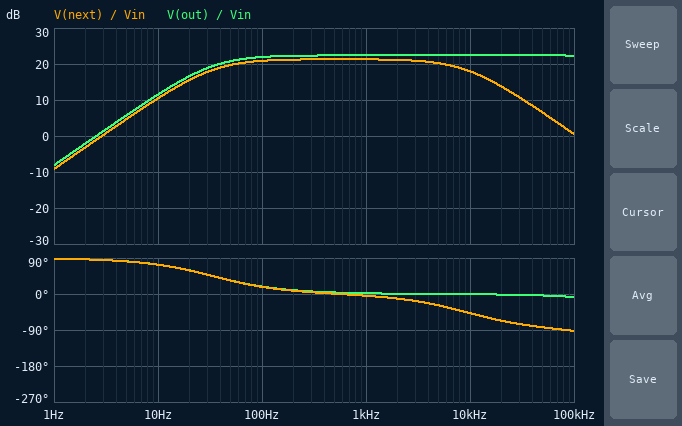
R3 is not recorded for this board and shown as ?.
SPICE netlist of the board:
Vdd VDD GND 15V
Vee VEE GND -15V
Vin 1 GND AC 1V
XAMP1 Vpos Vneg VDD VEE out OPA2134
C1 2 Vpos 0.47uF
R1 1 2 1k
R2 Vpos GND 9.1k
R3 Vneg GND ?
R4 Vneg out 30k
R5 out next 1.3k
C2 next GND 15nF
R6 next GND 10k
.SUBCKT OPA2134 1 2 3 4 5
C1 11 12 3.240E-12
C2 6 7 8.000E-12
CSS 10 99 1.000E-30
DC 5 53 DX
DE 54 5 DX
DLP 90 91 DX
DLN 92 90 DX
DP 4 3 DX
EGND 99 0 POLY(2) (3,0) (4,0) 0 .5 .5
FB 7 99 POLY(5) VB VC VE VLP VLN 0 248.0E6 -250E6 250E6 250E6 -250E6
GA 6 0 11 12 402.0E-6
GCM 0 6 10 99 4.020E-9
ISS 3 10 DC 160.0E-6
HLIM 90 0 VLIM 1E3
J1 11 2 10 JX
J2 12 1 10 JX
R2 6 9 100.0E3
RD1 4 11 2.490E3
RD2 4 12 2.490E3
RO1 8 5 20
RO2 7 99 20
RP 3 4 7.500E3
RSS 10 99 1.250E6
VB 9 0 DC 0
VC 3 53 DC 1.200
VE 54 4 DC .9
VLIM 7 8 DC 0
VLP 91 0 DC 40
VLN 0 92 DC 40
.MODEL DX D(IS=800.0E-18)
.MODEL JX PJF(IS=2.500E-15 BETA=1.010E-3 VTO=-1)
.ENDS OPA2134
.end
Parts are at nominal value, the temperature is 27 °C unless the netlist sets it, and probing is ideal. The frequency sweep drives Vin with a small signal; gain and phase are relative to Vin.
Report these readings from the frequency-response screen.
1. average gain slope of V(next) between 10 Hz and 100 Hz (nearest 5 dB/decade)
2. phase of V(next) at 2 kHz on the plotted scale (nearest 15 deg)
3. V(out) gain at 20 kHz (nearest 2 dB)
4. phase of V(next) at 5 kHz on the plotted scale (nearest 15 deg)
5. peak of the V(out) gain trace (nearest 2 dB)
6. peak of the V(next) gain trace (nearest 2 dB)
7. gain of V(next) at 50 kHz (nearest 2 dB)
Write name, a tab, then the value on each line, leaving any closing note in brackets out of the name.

average gain slope of V(next) between 10 Hz and 100 Hz	10 dB/decade
phase of V(next) at 2 kHz on the plotted scale	-15 deg
V(out) gain at 20 kHz	22 dB
phase of V(next) at 5 kHz on the plotted scale	-30 deg
peak of the V(out) gain trace	22 dB
peak of the V(next) gain trace	22 dB
gain of V(next) at 50 kHz	6 dB
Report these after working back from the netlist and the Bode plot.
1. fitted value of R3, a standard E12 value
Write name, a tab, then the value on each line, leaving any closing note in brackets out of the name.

fitted value of R3, a standard E12 value	2.2 kΩ
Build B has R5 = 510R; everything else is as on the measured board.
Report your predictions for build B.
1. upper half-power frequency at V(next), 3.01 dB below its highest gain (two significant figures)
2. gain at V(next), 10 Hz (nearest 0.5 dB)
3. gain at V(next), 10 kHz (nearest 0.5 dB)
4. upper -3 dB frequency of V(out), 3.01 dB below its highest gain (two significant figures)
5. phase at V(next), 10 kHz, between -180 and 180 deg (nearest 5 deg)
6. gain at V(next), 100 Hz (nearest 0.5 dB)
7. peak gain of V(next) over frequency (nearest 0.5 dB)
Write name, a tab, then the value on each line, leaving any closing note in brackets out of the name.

upper half-power frequency at V(next), 3.01 dB below its highest gain	22 kHz
gain at V(next), 10 Hz	11.0 dB
gain at V(next), 10 kHz	21.0 dB
upper -3 dB frequency of V(out), 3.01 dB below its highest gain	810 kHz
phase at V(next), 10 kHz, between -180 and 180 deg	-25 deg
gain at V(next), 100 Hz	21.5 dB
peak gain of V(next) over frequency	22.0 dB
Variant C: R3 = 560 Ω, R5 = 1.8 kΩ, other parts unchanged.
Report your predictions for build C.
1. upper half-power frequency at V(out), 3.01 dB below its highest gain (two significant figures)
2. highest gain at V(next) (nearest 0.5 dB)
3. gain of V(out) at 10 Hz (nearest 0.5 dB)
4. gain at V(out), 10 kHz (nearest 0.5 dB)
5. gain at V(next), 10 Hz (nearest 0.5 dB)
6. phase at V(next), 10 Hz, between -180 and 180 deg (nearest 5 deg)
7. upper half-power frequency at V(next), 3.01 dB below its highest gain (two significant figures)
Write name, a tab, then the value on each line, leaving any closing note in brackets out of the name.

upper half-power frequency at V(out), 3.01 dB below its highest gain	210 kHz
highest gain at V(next)	32.5 dB
gain of V(out) at 10 Hz	23.0 dB
gain at V(out), 10 kHz	34.0 dB
gain at V(next), 10 Hz	21.5 dB
phase at V(next), 10 Hz, between -180 and 180 deg	75 deg
upper half-power frequency at V(next), 3.01 dB below its highest gain	7.0 kHz
